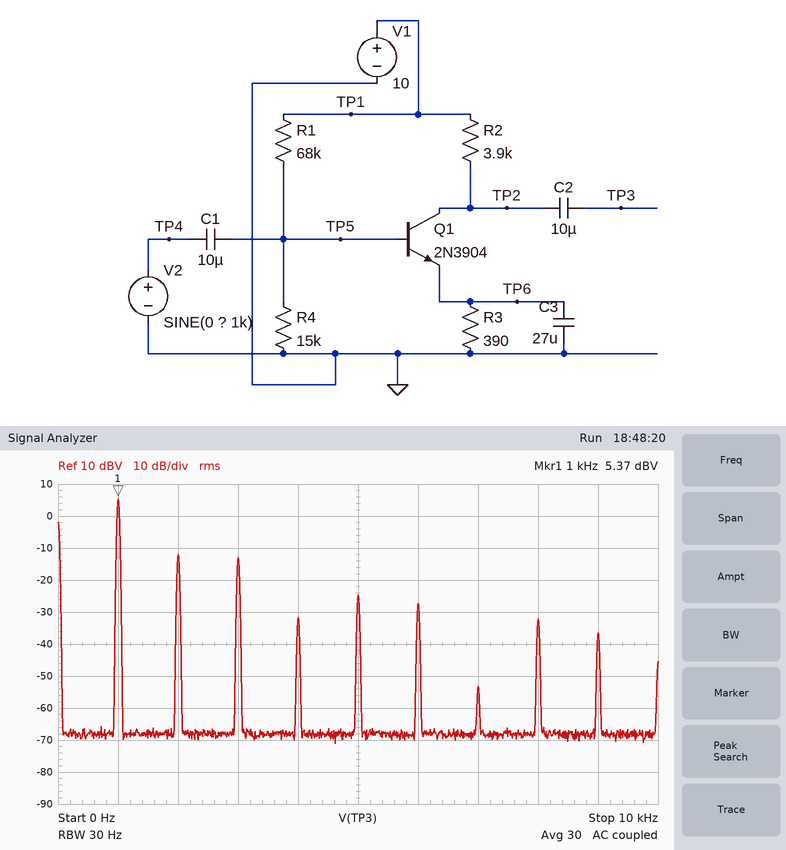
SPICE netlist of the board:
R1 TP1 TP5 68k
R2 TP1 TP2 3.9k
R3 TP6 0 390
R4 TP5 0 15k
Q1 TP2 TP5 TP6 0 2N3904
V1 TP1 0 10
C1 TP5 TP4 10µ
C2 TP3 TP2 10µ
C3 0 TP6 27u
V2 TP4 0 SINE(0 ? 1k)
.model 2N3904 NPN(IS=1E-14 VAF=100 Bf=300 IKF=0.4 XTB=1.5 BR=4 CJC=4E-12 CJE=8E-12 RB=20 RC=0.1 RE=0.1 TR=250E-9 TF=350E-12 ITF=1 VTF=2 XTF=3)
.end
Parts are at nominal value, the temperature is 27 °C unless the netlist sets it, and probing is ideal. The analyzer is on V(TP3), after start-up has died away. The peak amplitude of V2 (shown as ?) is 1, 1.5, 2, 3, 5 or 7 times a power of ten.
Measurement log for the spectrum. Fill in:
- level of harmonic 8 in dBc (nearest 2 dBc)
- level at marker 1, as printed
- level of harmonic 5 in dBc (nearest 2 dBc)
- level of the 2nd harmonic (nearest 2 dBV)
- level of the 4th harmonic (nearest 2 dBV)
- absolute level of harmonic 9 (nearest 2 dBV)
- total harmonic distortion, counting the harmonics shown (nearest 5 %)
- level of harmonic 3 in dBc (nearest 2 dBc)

-38 dBc
5.37 dBV
-30 dBc
-12 dBV
-32 dBV
-36 dBV
20 %
-18 dBc
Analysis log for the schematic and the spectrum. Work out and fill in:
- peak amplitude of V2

15 mV
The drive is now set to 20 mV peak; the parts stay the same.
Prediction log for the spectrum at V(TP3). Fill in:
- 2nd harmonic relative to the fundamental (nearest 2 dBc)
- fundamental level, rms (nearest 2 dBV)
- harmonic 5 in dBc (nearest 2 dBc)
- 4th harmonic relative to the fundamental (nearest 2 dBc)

-22 dBc
8 dBV
-32 dBc
-30 dBc
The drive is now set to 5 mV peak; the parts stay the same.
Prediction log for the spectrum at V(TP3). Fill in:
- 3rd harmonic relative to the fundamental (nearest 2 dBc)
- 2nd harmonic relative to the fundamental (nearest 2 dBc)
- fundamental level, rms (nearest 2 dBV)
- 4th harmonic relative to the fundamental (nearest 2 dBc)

-24 dBc
-10 dBc
-4 dBV
-26 dBc
